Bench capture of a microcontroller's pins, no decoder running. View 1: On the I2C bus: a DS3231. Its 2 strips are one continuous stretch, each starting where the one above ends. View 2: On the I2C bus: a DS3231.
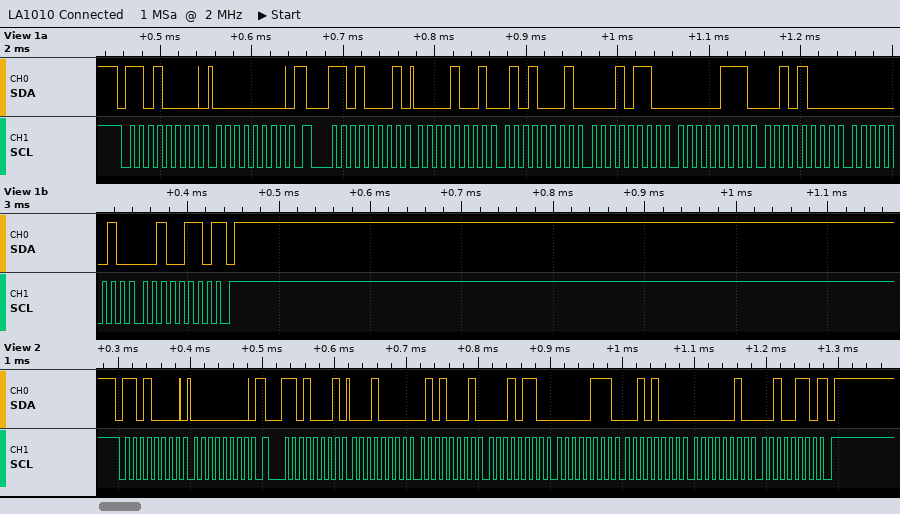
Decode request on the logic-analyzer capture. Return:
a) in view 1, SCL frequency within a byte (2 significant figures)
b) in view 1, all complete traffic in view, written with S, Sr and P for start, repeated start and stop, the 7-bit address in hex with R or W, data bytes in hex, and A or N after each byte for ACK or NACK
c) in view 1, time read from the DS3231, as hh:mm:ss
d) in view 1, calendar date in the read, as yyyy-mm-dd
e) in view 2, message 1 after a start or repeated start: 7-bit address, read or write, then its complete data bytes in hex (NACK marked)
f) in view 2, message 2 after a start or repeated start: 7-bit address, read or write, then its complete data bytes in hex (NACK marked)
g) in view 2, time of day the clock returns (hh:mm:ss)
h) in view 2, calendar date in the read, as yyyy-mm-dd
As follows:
100 kHz
S 68W A 00 A Sr 68R A 09 A 51 A 16 A 07 A 28 A 02 A 26 N P
16:51:09
2026-02-28
0x68 write: 00
0x68 read: 10 51 16 07 28 02 26 NACK
16:51:10
2026-02-28
